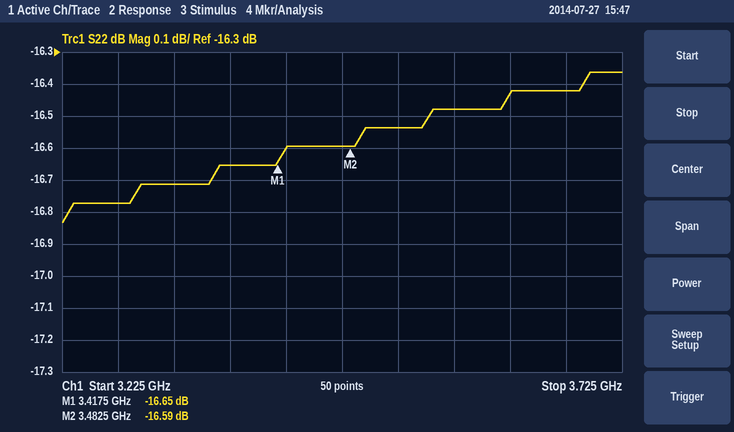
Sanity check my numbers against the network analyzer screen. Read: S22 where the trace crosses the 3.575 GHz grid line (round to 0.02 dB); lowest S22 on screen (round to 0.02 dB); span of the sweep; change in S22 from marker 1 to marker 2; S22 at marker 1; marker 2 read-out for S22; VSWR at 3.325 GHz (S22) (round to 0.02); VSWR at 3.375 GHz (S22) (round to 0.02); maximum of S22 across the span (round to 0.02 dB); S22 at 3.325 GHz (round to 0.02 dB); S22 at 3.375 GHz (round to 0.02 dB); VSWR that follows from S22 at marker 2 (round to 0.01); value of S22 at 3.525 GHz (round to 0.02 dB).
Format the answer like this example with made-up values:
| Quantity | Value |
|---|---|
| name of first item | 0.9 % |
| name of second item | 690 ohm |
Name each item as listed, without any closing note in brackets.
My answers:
| Quantity | Value |
|---|---|
| S22 where the trace crosses the 3.575 GHz grid line | -16.48 dB |
| lowest S22 on screen | -16.84 dB |
| span of the sweep | 500 MHz |
| change in S22 from marker 1 to marker 2 | 0.06 dB |
| S22 at marker 1 | -16.65 dB |
| marker 2 read-out for S22 | -16.59 dB |
| VSWR at 3.325 GHz (S22) | 1.34 |
| VSWR at 3.375 GHz (S22) | 1.34 |
| maximum of S22 across the span | -16.36 dB |
| S22 at 3.325 GHz | -16.72 dB |
| S22 at 3.375 GHz | -16.66 dB |
| VSWR that follows from S22 at marker 2 | 1.35 |
| value of S22 at 3.525 GHz | -16.54 dB |
